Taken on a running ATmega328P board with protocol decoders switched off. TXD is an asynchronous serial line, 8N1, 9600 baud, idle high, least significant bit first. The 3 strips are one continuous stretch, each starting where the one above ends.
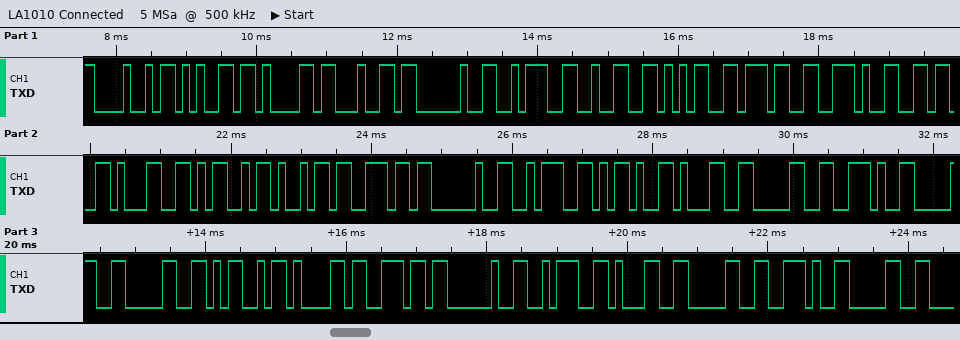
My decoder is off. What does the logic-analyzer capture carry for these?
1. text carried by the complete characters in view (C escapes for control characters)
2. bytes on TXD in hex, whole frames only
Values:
"Head :257.61Min :-10.00Man :10.0"
48 65 61 64 20 3A 32 35 37 2E 36 31 4D 69 6E 20 3A 2D 31 30 2E 30 30 4D 61 6E 20 3A 31 30 2E 30
